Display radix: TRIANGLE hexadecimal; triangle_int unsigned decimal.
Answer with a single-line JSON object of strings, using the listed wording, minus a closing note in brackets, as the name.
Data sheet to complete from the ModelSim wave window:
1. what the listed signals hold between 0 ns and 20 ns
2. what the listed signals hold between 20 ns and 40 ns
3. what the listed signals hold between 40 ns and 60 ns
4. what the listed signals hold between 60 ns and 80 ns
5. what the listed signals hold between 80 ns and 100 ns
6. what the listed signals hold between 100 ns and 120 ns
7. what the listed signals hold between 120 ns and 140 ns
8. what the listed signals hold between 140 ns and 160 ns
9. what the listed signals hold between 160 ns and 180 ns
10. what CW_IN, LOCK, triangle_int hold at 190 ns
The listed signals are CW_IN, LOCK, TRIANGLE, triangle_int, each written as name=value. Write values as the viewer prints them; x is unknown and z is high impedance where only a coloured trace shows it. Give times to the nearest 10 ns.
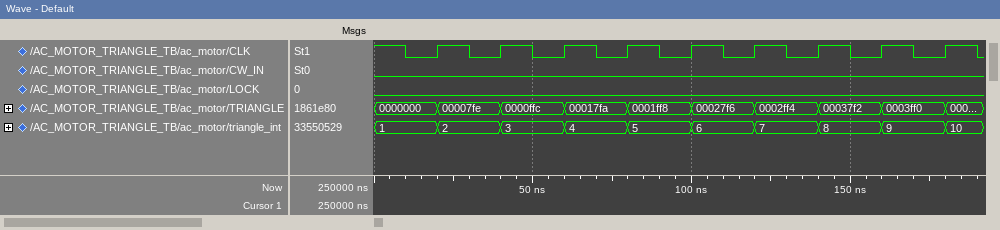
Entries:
{"what the listed signals hold between 0 ns and 20 ns": "CW_IN=0, LOCK=0, TRIANGLE=0000000, triangle_int=1", "what the listed signals hold between 20 ns and 40 ns": "CW_IN=0, LOCK=0, TRIANGLE=00007fe, triangle_int=2", "what the listed signals hold between 40 ns and 60 ns": "CW_IN=0, LOCK=0, TRIANGLE=0000ffc, triangle_int=3", "what the listed signals hold between 60 ns and 80 ns": "CW_IN=0, LOCK=0, TRIANGLE=00017fa, triangle_int=4", "what the listed signals hold between 80 ns and 100 ns": "CW_IN=0, LOCK=0, TRIANGLE=0001ff8, triangle_int=5", "what the listed signals hold between 100 ns and 120 ns": "CW_IN=0, LOCK=0, TRIANGLE=00027f6, triangle_int=6", "what the listed signals hold between 120 ns and 140 ns": "CW_IN=0, LOCK=0, TRIANGLE=0002ff4, triangle_int=7", "what the listed signals hold between 140 ns and 160 ns": "CW_IN=0, LOCK=0, TRIANGLE=00037f2, triangle_int=8", "what the listed signals hold between 160 ns and 180 ns": "CW_IN=0, LOCK=0, TRIANGLE=0003ff0, triangle_int=9", "what CW_IN, LOCK, triangle_int hold at 190 ns": "CW_IN=0, LOCK=0, triangle_int=10"}
